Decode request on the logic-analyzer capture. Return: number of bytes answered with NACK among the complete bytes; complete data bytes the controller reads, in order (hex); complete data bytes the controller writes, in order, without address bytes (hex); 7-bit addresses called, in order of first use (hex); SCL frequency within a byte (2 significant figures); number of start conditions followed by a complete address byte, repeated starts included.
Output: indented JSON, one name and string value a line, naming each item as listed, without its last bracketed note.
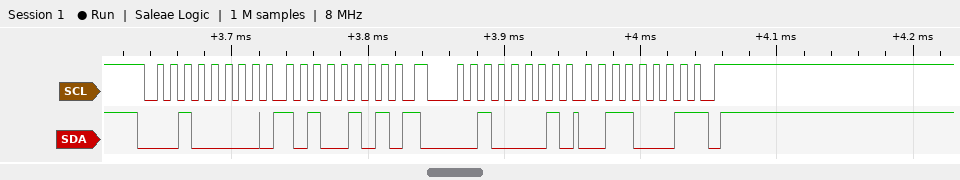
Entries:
{
  "number of bytes answered with NACK among the complete bytes": "1",
  "complete data bytes the controller reads, in order": "31",
  "complete data bytes the controller writes, in order, without address bytes": "A5",
  "7-bit addresses called, in order of first use": "0x10",
  "SCL frequency within a byte": "100 kHz",
  "number of start conditions followed by a complete address byte, repeated starts included": "2"
}
